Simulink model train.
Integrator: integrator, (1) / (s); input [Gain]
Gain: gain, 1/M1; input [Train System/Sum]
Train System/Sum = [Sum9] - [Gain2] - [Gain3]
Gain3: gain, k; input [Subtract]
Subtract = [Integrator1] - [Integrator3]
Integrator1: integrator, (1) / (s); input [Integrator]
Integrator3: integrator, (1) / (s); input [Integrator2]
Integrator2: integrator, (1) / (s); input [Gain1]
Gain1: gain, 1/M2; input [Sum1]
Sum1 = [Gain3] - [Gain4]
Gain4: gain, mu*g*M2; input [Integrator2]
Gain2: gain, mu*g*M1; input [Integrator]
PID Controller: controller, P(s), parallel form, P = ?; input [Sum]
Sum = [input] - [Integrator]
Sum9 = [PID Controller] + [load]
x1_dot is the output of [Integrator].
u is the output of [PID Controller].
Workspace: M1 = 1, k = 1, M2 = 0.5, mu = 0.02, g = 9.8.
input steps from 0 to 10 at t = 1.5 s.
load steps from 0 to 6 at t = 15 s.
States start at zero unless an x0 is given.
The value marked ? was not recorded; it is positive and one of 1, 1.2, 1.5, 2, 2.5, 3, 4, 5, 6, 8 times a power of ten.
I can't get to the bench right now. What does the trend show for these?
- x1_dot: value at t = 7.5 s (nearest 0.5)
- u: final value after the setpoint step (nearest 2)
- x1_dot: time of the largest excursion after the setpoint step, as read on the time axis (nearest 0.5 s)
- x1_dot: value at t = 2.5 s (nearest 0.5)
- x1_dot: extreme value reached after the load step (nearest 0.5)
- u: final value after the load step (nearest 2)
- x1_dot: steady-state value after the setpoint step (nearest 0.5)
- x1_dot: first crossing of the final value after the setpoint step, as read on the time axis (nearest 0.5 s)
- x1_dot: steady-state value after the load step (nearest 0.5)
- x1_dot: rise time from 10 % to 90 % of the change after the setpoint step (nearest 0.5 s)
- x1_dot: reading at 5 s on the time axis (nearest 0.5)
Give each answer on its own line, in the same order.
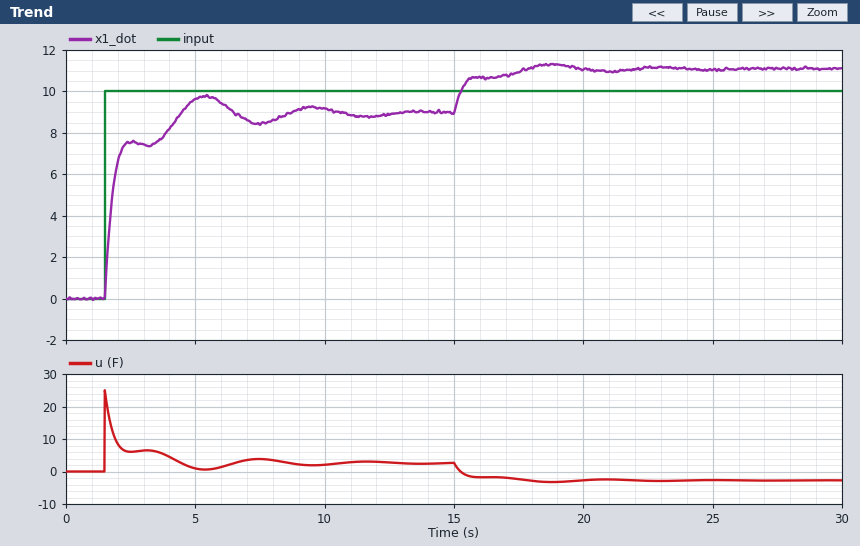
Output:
8.5
2
5.5 s
7.5
11.5
-2
9.0
4.5 s
11.0
2.5 s
9.5
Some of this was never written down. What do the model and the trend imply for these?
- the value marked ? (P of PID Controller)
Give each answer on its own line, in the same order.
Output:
2.5
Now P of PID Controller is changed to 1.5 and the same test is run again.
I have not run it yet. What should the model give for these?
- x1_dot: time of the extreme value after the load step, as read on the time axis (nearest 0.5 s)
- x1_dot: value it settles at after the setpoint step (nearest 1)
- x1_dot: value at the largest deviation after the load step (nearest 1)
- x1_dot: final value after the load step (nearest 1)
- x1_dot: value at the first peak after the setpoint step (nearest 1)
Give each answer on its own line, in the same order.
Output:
19.0 s
8
12
12
9
